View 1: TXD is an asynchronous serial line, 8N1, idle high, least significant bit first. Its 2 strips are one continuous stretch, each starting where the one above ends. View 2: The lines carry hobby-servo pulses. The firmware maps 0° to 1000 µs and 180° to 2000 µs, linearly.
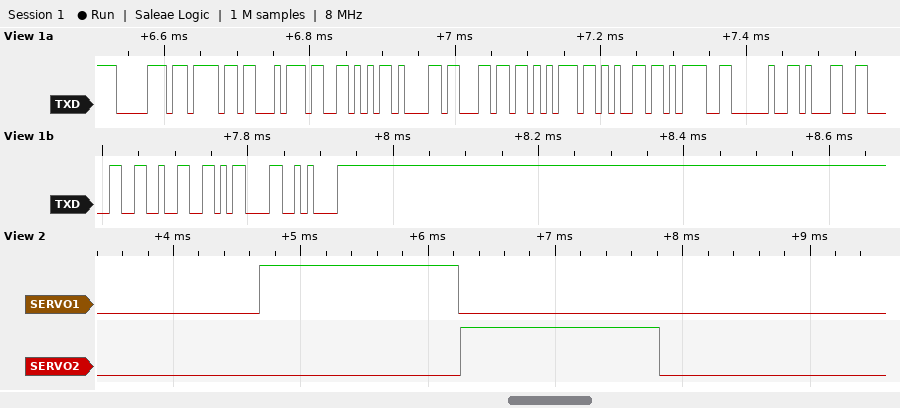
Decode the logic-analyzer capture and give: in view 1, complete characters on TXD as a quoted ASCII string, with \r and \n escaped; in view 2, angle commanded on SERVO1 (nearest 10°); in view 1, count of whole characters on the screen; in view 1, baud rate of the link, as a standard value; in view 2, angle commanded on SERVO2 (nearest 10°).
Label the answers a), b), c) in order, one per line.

a) "potValue= 102\r\n"
b) 100°
c) 15
d) 115200 baud
e) 100°
